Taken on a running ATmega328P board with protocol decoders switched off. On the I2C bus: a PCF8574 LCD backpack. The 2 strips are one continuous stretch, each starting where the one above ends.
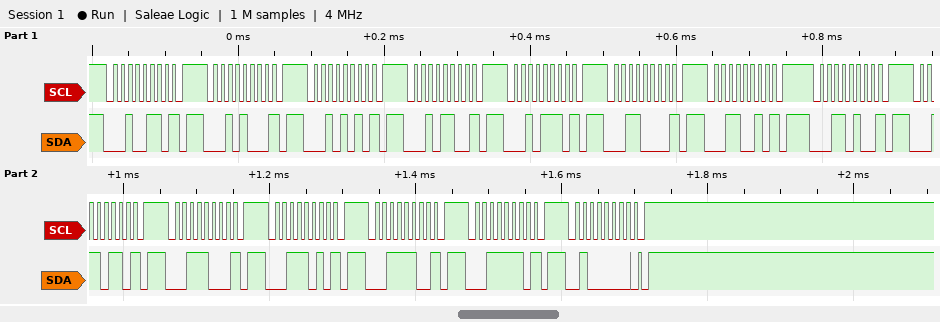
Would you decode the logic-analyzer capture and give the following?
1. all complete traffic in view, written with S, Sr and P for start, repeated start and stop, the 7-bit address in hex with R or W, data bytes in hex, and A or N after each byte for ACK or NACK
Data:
S 13W N P S 14W N P S 15W N P S 16W N P S 17W N P S 18W N P S 19W N P S 1AW N P S 1BW N P S 1CW N P S 1DW N P S 1EW N P S 1FW N P S 20W A P
